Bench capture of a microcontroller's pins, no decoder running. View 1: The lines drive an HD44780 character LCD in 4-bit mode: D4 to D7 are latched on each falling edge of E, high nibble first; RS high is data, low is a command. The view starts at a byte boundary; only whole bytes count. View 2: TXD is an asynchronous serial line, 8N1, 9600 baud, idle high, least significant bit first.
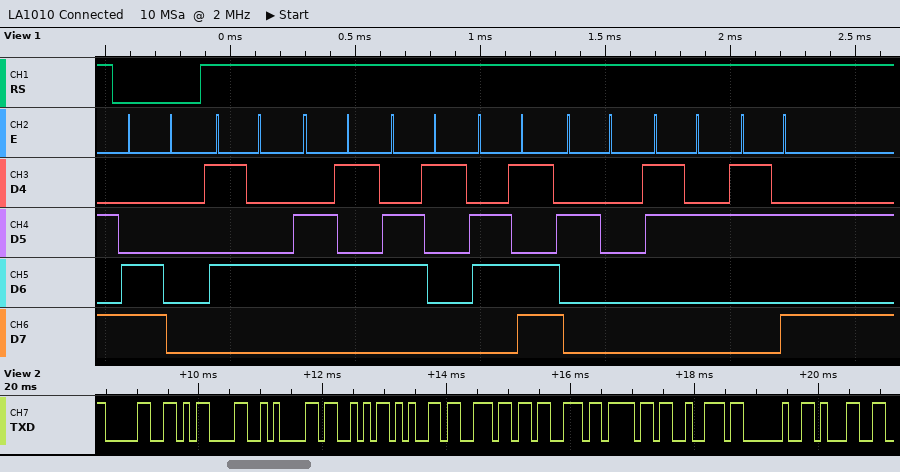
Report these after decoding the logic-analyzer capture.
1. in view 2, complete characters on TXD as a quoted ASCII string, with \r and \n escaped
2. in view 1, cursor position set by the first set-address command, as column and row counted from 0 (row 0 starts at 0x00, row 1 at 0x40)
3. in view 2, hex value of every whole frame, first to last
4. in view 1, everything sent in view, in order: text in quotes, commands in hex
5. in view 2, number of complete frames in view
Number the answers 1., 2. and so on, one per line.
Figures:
1. "0\r\nSensor 1"
2. column 0, row 1
3. 0x30 0x0D 0x0A 0x53 0x65 0x6E 0x73 0x6F 0x72 0x20 0x31
4. 0xC0 "Team 2:"
5. 11
